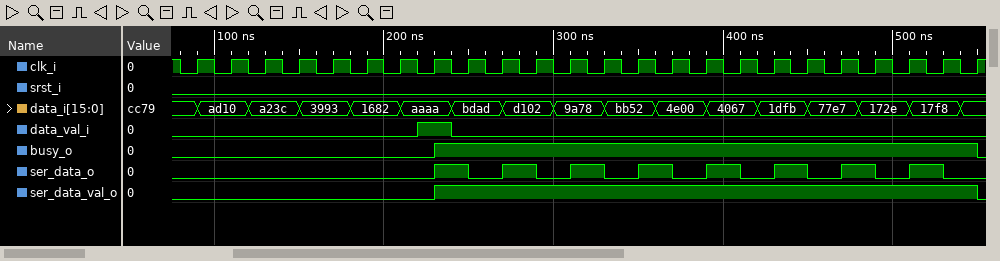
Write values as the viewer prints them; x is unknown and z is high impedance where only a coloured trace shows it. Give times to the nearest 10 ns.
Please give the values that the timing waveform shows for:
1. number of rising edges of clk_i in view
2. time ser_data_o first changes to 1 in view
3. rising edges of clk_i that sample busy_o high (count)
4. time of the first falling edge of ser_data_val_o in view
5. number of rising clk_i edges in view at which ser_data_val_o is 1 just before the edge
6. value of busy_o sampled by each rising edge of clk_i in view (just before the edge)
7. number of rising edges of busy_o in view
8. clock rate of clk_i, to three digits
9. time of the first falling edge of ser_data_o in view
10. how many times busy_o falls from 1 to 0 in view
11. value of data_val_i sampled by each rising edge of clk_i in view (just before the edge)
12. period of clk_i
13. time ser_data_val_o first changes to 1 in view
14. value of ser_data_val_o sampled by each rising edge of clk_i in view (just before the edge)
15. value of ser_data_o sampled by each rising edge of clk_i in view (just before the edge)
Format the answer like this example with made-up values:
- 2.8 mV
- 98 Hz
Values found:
- 24
- 230 ns
- 16
- 550 ns
- 16
- 0 0 0 0 0 0 0 0 1 1 1 1 1 1 1 1 1 1 1 1 1 1 1 1
- 1
- 50.0 MHz
- 250 ns
- 1
- 0 0 0 0 0 0 0 1 0 0 0 0 0 0 0 0 0 0 0 0 0 0 0 0
- 20 ns
- 230 ns
- 0 0 0 0 0 0 0 0 1 1 1 1 1 1 1 1 1 1 1 1 1 1 1 1
- 0 0 0 0 0 0 0 0 1 0 1 0 1 0 1 0 1 0 1 0 1 0 1 0
